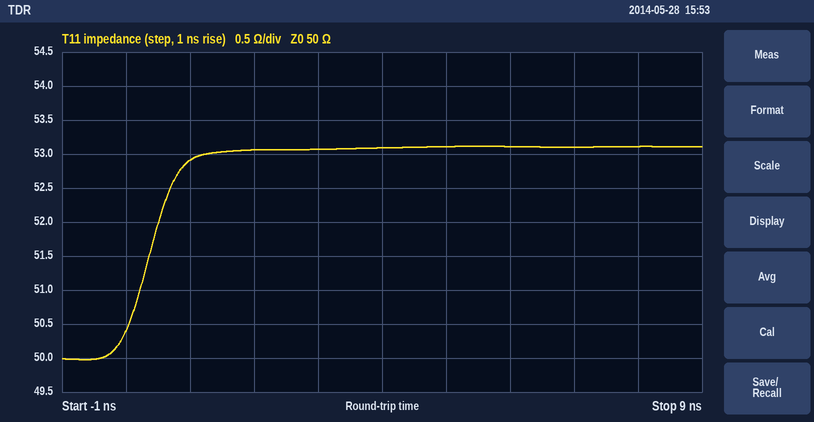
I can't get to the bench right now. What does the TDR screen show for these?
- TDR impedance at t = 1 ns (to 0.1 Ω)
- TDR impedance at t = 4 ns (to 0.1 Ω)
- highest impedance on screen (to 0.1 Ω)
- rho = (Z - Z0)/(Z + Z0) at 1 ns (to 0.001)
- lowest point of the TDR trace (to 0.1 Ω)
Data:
52.9 Ω
53.1 Ω
53.1 Ω
+0.028
50.0 Ω
